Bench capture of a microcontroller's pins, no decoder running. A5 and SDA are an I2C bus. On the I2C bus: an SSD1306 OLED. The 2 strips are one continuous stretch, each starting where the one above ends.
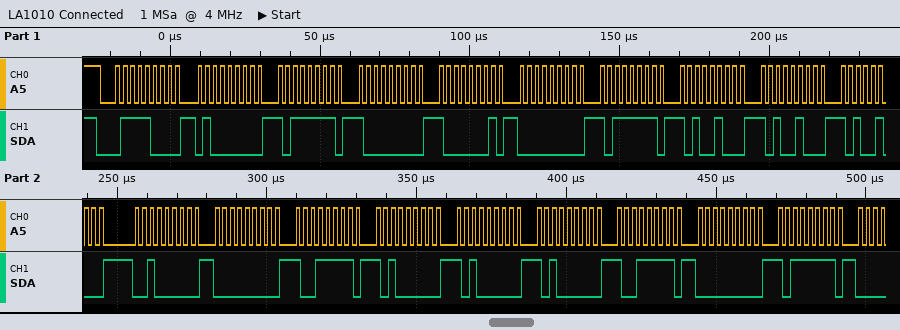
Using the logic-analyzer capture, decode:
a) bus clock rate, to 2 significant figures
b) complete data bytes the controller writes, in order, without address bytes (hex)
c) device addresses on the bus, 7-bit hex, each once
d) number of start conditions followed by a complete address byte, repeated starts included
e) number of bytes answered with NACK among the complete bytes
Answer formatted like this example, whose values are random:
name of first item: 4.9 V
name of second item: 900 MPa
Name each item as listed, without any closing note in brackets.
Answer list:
bus clock rate, to 2 significant figures: 400 kHz
complete data bytes the controller writes, in order, without address bytes: 40 BF 80 81 00 BF A4 A4 A4 20 00 9F A0 A0 A0 9F 00 BF
device addresses on the bus, 7-bit hex, each once: 0x3C
number of start conditions followed by a complete address byte, repeated starts included: 1
number of bytes answered with NACK among the complete bytes: 0
